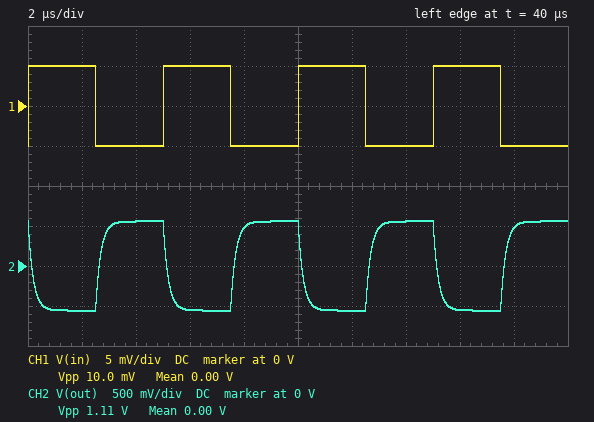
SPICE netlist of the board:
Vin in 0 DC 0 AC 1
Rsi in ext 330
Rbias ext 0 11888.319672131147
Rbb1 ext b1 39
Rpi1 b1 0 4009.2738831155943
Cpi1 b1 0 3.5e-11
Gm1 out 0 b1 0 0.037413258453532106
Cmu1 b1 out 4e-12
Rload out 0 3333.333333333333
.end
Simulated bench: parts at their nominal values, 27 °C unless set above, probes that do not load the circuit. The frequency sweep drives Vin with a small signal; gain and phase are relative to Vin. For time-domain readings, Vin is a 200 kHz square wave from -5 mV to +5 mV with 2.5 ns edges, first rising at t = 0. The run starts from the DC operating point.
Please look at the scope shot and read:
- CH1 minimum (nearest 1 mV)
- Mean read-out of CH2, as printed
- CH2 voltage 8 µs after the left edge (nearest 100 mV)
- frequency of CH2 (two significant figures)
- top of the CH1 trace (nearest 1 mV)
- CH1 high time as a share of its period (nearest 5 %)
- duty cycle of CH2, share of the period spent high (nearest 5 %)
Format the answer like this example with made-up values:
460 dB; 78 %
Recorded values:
-5 mV; 0.00 V; 500 mV; 200 kHz; 5 mV; 50 %; 50 %
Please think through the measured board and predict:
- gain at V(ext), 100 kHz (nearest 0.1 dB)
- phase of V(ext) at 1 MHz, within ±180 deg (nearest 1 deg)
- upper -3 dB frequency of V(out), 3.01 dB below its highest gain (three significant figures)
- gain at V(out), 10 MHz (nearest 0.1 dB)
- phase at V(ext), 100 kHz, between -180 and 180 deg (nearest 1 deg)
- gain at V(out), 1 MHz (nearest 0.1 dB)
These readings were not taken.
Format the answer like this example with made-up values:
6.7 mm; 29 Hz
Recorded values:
-1.0 dB; -38 deg; 837 kHz; 19.3 dB; -6 deg; 37.1 dB
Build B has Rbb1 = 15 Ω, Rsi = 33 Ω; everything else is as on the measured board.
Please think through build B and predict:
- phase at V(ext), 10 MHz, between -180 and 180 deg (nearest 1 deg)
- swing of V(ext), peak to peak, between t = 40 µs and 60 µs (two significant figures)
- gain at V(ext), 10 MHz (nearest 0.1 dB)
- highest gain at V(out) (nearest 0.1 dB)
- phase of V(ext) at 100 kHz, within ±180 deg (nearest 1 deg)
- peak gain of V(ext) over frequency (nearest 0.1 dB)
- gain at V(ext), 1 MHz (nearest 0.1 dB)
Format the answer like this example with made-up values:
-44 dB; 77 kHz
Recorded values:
-15 deg; 9.9 mV; -4.0 dB; 41.8 dB; -1 deg; -0.1 dB; -0.3 dB
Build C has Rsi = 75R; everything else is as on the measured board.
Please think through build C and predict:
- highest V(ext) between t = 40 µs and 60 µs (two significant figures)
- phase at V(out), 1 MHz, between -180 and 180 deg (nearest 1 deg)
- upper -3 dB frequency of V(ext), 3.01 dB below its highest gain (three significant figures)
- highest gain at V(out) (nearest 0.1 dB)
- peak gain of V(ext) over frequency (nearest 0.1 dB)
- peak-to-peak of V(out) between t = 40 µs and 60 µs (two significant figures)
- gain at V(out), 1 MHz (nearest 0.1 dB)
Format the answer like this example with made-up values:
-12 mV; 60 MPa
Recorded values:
4.9 mV; 155 deg; 2.94 MHz; 41.6 dB; -0.2 dB; 1.2 V; 40.8 dB
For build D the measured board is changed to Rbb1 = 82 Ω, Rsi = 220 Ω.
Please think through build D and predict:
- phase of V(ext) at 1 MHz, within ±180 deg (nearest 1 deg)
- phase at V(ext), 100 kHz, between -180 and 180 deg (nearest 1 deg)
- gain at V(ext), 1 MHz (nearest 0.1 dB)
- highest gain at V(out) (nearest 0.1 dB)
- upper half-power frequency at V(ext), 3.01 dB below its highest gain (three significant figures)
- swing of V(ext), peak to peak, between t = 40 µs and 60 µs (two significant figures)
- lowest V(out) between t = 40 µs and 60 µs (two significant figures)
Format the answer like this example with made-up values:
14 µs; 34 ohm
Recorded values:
-26 deg; -4 deg; -3.2 dB; 41.1 dB; 1.13 MHz; 9.3 mV; -570 mV
